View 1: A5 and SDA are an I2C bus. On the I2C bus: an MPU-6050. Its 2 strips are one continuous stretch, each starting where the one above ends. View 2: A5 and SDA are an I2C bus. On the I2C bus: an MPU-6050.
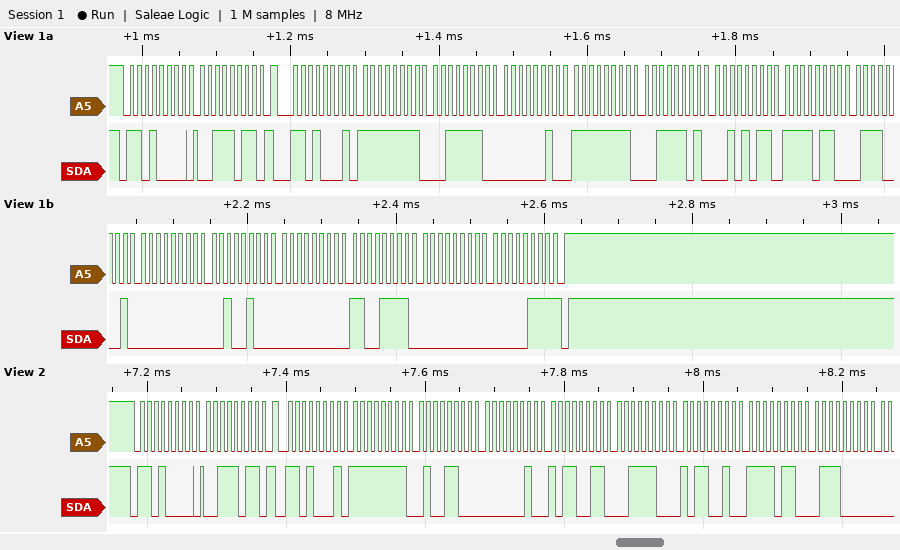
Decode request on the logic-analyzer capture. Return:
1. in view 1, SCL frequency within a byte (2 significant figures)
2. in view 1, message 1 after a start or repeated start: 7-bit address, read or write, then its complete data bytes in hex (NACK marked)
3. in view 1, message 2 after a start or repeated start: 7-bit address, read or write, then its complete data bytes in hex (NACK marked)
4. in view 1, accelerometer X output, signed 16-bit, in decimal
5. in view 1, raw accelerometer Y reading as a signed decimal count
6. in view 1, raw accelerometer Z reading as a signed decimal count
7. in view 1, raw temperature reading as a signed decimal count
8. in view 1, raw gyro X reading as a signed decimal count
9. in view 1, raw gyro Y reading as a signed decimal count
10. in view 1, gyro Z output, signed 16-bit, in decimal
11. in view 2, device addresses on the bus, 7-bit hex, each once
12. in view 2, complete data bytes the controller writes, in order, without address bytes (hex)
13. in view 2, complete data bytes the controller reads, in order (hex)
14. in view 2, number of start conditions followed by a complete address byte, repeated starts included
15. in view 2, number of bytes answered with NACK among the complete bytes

100 kHz
0x68 write: 3B
0x68 read: FF 3E 02 FF 3D 2B F6 71 00 24 00 CF 00 07 NACK
-194
767
15659
-2447
36
207
7
0x68
3B
FF 4C 02 B3 3C B2 F6 70
2
0
